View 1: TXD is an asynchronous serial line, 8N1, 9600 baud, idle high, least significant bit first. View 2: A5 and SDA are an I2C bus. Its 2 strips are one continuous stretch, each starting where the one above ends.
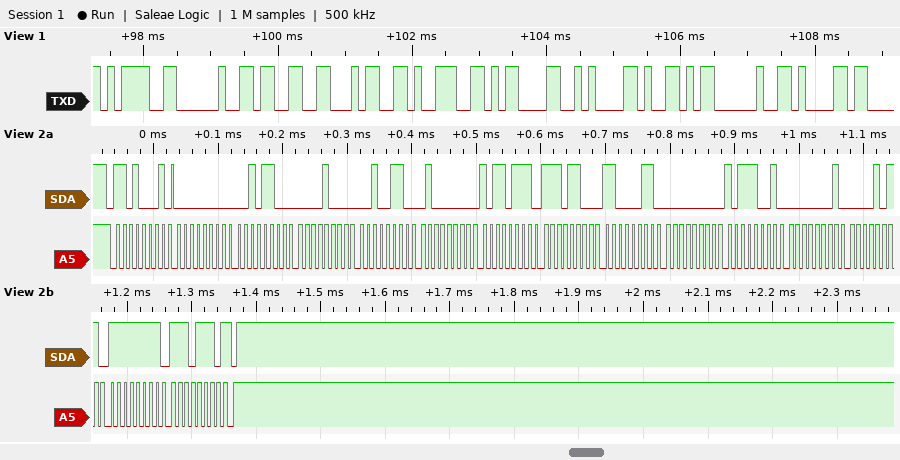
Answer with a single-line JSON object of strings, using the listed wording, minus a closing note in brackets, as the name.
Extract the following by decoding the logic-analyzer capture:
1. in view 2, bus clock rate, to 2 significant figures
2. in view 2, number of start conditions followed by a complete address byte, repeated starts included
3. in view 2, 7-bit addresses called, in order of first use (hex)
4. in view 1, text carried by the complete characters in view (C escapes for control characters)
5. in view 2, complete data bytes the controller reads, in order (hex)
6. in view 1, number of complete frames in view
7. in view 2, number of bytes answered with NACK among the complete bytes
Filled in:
{"in view 2, bus clock rate, to 2 significant figures": "100 kHz", "in view 2, number of start conditions followed by a complete address byte, repeated starts included": "1", "in view 2, 7-bit addresses called, in order of first use": "0x68", "in view 1, text carried by the complete characters in view": "\"= 349\\r\\nY a\"", "in view 2, complete data bytes the controller reads, in order": "00 2C 08 26 40 B7 EC C3 00 B9 01 0B FF EE", "in view 1, number of complete frames in view": "10", "in view 2, number of bytes answered with NACK among the complete bytes": "1"}
